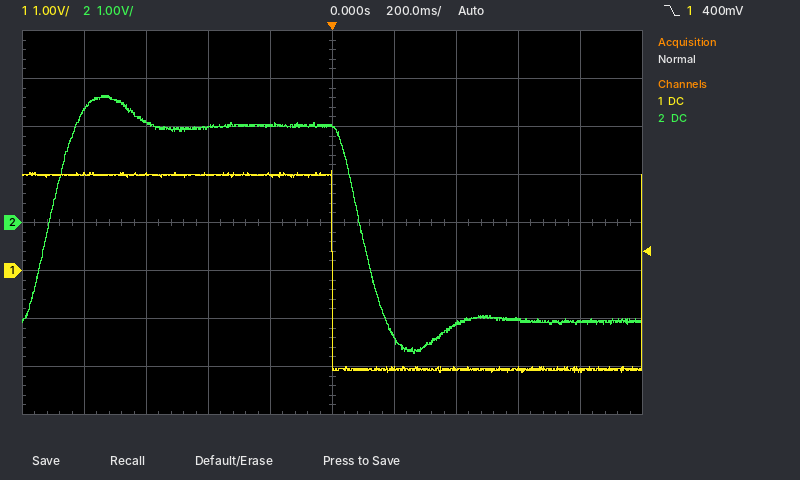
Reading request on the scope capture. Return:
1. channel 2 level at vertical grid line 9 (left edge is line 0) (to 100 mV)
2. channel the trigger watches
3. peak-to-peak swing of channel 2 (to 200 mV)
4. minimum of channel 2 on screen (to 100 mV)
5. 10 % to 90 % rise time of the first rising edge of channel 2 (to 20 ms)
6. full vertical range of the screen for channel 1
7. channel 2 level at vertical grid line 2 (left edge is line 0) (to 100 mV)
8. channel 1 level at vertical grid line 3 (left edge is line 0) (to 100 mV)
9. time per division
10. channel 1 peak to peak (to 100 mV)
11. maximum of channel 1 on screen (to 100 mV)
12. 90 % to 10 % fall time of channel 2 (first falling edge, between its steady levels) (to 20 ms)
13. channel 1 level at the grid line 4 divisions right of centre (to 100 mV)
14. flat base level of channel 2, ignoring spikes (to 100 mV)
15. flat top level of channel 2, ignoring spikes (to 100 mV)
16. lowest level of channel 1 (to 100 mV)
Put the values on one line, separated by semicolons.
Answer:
-2.1 V; channel 1; 5.4 V; -2.7 V; 120 ms; 8 V; 2.1 V; 2.0 V; 200 ms; 4.2 V; 2.1 V; 120 ms; -2.1 V; -2.1 V; 2.0 V; -2.1 V
